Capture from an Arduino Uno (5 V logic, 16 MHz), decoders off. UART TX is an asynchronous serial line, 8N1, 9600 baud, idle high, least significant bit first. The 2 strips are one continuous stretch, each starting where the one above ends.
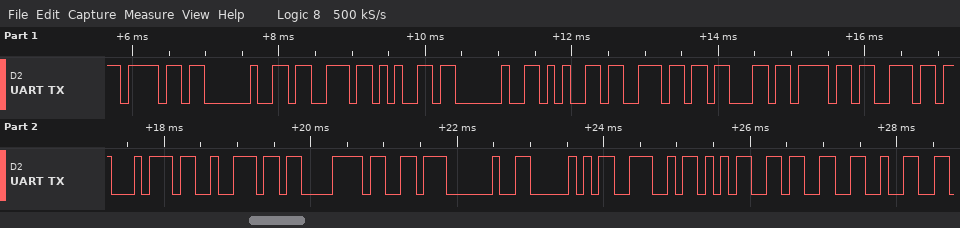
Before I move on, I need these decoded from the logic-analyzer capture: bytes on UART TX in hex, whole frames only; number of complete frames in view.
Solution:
6F 20 73 65 20 65 6E 63 6F 6E 74 72 C3 B3 20 50 4E 35 33 32
20
